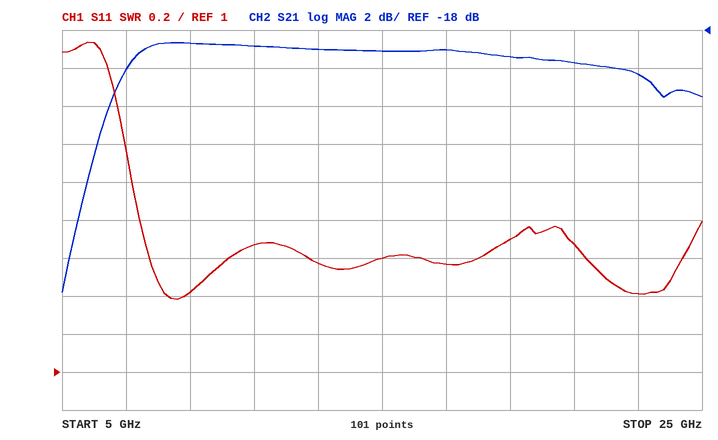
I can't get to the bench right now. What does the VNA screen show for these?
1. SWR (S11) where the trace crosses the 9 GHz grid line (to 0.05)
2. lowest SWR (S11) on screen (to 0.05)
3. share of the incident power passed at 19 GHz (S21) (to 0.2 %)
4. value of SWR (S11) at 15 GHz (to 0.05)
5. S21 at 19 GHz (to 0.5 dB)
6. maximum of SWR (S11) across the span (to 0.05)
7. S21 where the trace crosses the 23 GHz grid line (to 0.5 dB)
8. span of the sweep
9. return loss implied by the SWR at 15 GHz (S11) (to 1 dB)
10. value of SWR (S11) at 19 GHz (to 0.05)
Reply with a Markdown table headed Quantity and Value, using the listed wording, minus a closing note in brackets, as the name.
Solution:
| Quantity | Value |
|---|---|
| SWR (S11) where the trace crosses the 9 GHz grid line | 1.40 |
| lowest SWR (S11) on screen | 1.40 |
| share of the incident power passed at 19 GHz (S21) | 1.2 % |
| value of SWR (S11) at 15 GHz | 1.60 |
| S21 at 19 GHz | -19.5 dB |
| maximum of SWR (S11) across the span | 2.75 |
| S21 where the trace crosses the 23 GHz grid line | -20.5 dB |
| span of the sweep | 20 GHz |
| return loss implied by the SWR at 15 GHz (S11) | 13 dB |
| value of SWR (S11) at 19 GHz | 1.70 |
